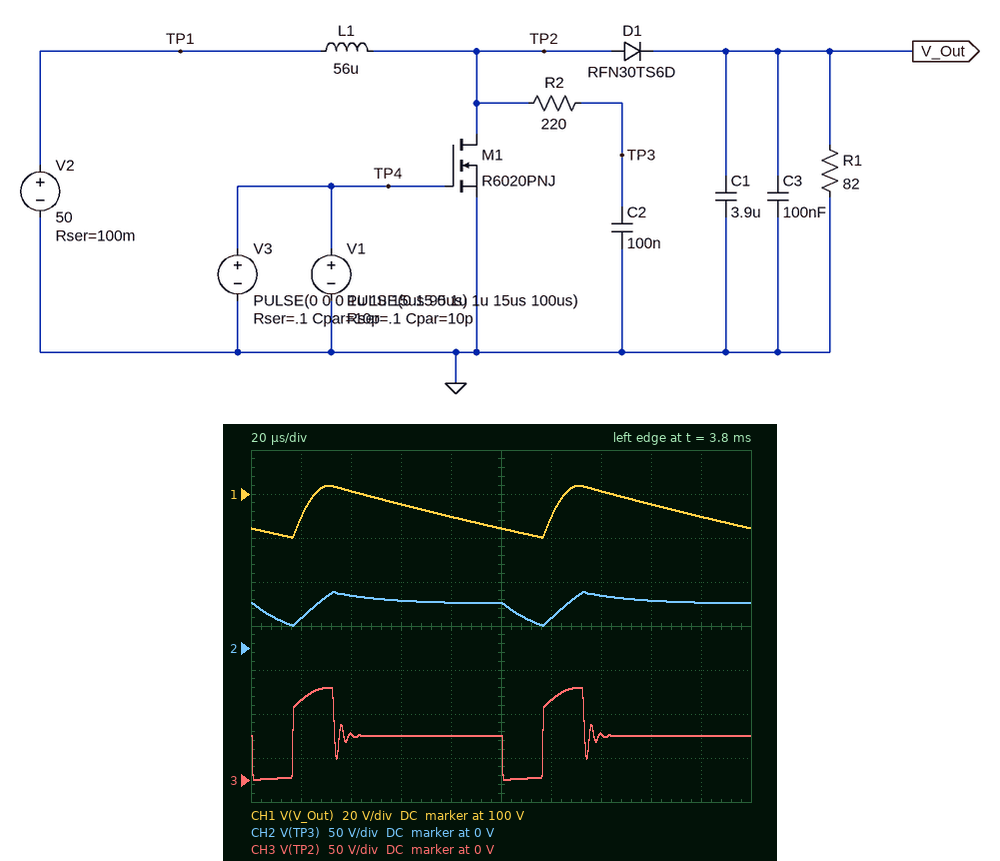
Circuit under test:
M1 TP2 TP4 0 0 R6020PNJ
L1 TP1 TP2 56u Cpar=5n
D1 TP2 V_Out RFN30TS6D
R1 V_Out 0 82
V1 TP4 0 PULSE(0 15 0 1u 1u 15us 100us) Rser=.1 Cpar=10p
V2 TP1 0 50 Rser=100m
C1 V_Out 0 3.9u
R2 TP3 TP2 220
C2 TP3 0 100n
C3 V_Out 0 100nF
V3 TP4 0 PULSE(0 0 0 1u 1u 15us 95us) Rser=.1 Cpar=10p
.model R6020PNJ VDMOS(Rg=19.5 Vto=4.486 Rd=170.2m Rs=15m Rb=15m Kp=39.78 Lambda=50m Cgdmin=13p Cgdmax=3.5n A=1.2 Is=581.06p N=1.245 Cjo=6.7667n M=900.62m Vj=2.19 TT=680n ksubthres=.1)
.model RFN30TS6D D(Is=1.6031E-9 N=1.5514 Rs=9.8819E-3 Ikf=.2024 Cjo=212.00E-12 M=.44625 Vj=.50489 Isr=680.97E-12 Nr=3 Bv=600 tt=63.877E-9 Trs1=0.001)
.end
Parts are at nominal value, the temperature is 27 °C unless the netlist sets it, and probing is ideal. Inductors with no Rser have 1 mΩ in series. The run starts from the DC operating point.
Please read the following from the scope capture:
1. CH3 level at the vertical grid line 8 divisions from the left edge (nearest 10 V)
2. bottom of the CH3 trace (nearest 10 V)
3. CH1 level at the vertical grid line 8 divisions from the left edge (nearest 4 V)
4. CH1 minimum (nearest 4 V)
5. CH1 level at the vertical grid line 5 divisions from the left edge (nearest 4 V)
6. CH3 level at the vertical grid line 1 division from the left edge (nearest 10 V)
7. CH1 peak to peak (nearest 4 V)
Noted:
50 V
0 V
96 V
80 V
84 V
90 V
24 V
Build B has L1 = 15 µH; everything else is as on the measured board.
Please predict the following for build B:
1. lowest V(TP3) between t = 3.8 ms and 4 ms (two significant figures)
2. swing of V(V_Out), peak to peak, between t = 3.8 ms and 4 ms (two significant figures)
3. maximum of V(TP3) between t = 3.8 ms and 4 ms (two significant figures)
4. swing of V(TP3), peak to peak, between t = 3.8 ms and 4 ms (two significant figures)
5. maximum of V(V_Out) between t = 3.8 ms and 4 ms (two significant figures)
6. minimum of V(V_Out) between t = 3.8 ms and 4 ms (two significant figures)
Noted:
27 V
38 V
60 V
33 V
150 V
120 V
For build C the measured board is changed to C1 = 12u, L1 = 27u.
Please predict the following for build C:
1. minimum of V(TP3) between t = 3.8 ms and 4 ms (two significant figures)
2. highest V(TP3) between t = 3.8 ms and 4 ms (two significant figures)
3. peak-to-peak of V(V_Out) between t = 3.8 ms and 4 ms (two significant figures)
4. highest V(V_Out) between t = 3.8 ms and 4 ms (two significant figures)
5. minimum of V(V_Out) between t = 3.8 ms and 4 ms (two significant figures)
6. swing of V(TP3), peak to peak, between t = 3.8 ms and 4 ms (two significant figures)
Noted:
26 V
62 V
10 V
120 V
110 V
36 V
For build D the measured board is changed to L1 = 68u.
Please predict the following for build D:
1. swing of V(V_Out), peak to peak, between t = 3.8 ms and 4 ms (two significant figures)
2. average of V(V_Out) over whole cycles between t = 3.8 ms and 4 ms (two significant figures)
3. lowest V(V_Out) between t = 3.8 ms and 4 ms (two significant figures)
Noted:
22 V
87 V
76 V
